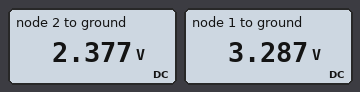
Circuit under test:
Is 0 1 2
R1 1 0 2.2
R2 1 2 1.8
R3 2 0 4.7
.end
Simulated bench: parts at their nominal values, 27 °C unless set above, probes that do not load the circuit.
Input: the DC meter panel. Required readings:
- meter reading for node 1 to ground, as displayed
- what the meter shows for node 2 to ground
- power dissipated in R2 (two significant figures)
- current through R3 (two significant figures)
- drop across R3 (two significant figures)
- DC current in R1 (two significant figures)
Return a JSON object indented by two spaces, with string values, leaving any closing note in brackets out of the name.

{
  "meter reading for node 1 to ground, as displayed": "3.287 V",
  "what the meter shows for node 2 to ground": "2.377 V",
  "power dissipated in R2": "460 mW",
  "current through R3": "510 mA",
  "drop across R3": "2.4 V",
  "DC current in R1": "1.5 A"
}
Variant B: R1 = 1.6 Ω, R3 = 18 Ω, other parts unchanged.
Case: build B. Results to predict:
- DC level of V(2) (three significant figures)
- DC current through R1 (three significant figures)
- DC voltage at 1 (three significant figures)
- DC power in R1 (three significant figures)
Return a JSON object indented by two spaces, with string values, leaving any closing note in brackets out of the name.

{
  "DC level of V(2)": "2.69 V",
  "DC current through R1": "1.85 A",
  "DC voltage at 1": "2.96 V",
  "DC power in R1": "5.48 W"
}
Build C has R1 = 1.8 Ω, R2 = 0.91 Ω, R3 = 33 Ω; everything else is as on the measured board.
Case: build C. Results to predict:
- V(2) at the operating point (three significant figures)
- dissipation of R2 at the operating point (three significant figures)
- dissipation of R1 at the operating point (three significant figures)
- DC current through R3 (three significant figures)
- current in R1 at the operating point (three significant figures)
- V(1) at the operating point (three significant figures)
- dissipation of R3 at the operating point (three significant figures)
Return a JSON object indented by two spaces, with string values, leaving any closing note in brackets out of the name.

{
  "V(2) at the operating point": "3.33 V",
  "dissipation of R2 at the operating point": "9.25 mW",
  "dissipation of R1 at the operating point": "6.49 W",
  "DC current through R3": "101 mA",
  "current in R1 at the operating point": "1.90 A",
  "V(1) at the operating point": "3.42 V",
  "dissipation of R3 at the operating point": "335 mW"
}
